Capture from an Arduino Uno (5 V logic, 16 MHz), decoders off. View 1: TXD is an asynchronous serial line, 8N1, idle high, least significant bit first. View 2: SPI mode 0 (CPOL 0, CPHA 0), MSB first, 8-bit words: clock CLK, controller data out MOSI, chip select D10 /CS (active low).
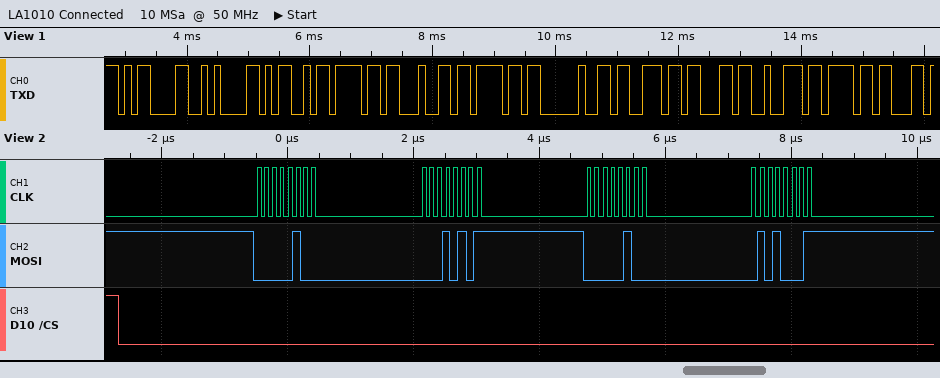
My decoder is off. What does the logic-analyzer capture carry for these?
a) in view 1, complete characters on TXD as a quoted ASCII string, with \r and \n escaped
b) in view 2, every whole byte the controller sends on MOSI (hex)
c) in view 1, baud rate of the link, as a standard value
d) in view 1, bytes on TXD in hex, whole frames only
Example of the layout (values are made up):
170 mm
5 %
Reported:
"\r\nModo scro"
04 15 04 51
9600 baud
0D 0A 4D 6F 64 6F 20 73 63 72 6F
